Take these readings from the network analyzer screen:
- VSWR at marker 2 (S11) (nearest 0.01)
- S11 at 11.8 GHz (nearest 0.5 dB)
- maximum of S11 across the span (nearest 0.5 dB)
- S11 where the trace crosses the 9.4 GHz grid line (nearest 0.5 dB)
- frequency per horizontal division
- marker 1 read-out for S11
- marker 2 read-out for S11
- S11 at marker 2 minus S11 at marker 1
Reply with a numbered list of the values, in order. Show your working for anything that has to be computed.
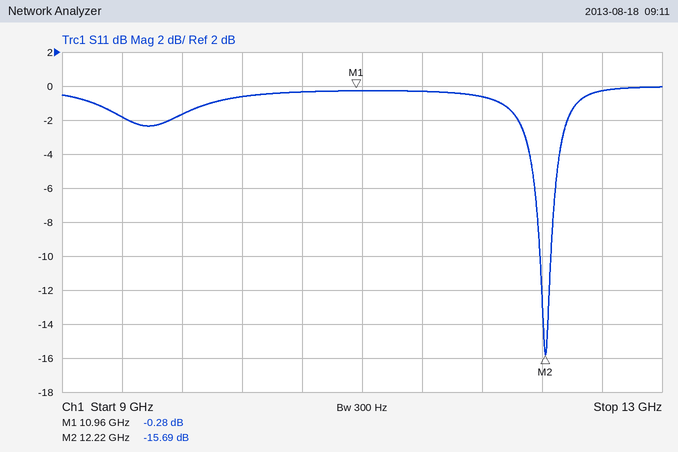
1. (1 + 0.1642)/(1 − 0.1642) ≈ 1.39
2. -0.5 dB
3. 0.0 dB
4. -2.0 dB
5. 400 MHz
6. -0.28 dB
7. -15.69 dB
8. -15.69 − (-0.28) = -15.41 dB
